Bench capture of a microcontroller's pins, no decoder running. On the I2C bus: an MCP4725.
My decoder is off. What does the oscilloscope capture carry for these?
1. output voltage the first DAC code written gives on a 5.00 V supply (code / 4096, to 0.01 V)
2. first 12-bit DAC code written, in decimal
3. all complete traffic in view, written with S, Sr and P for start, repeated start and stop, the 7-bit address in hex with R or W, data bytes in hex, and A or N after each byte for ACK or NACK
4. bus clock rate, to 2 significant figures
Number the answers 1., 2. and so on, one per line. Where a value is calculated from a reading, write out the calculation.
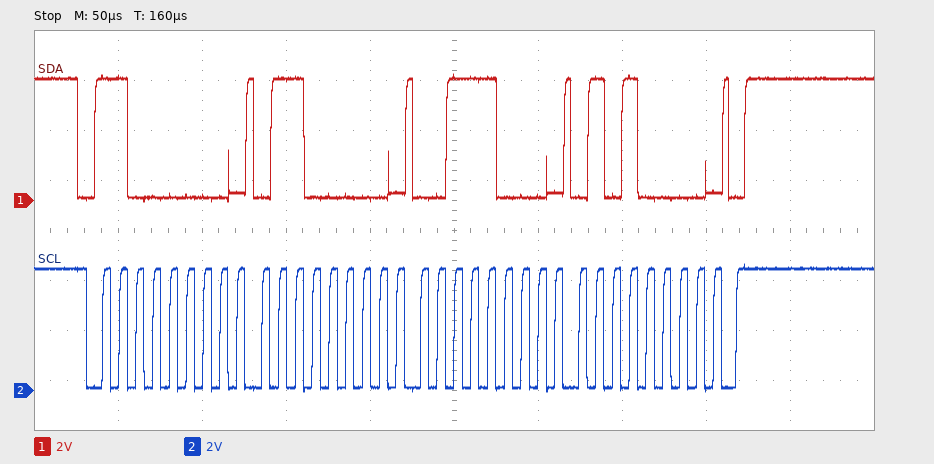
1. 901 / 4096 x 5.00 V = 1.10 V
2. 901
3. S 60W A 60 A 38 A 50 A P
4. 100 kHz
